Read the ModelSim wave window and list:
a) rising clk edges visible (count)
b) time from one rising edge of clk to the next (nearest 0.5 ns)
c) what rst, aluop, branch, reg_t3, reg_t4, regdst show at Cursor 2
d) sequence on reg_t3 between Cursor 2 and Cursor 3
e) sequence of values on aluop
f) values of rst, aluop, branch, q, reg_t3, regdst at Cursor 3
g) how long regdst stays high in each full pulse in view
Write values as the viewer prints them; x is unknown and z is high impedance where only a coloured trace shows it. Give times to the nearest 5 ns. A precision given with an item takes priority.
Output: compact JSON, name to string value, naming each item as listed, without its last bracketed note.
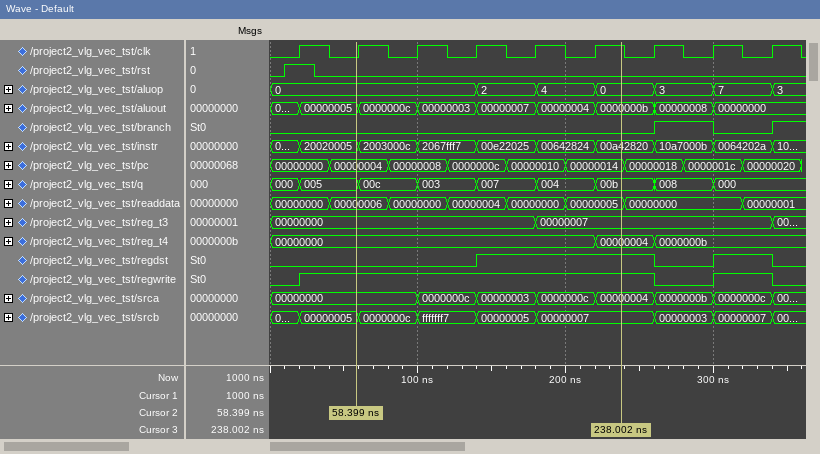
{"rising clk edges visible": "9", "time from one rising edge of clk to the next": "40 ns", "what rst, aluop, branch, reg_t3, reg_t4, regdst show at Cursor 2": "rst=0, aluop=0, branch=0, reg_t3=00000000, reg_t4=00000000, regdst=0", "sequence on reg_t3 between Cursor 2 and Cursor 3": "00000000, 00000007", "sequence of values on aluop": "0, 2, 4, 0, 3, 7, 3", "values of rst, aluop, branch, q, reg_t3, regdst at Cursor 3": "rst=0, aluop=0, branch=0, q=00b, reg_t3=00000007, regdst=1", "how long regdst stays high in each full pulse in view": "120 ns, 40 ns"}
